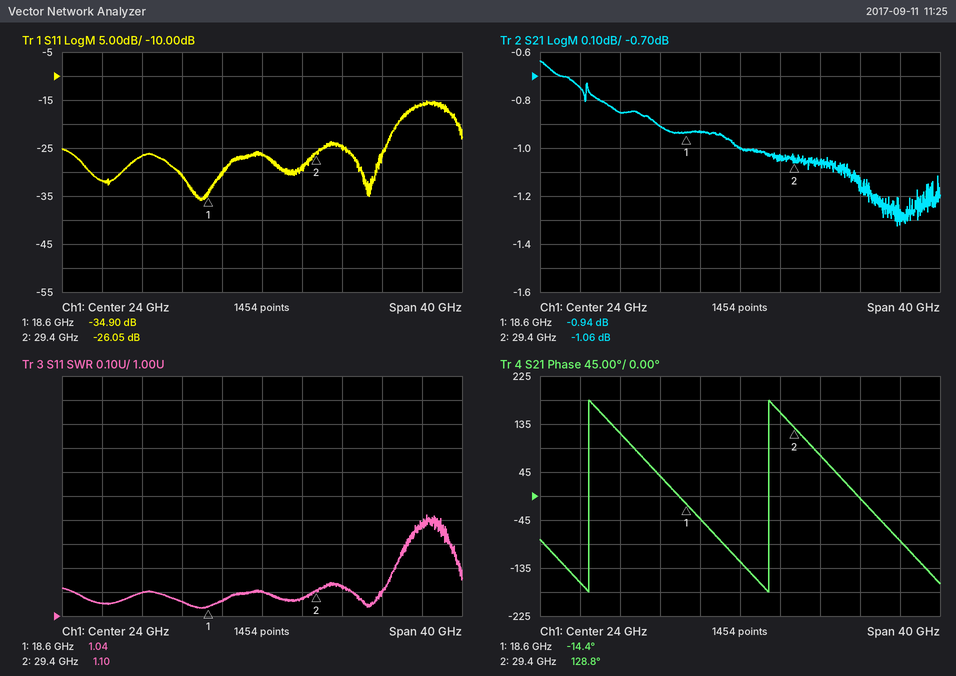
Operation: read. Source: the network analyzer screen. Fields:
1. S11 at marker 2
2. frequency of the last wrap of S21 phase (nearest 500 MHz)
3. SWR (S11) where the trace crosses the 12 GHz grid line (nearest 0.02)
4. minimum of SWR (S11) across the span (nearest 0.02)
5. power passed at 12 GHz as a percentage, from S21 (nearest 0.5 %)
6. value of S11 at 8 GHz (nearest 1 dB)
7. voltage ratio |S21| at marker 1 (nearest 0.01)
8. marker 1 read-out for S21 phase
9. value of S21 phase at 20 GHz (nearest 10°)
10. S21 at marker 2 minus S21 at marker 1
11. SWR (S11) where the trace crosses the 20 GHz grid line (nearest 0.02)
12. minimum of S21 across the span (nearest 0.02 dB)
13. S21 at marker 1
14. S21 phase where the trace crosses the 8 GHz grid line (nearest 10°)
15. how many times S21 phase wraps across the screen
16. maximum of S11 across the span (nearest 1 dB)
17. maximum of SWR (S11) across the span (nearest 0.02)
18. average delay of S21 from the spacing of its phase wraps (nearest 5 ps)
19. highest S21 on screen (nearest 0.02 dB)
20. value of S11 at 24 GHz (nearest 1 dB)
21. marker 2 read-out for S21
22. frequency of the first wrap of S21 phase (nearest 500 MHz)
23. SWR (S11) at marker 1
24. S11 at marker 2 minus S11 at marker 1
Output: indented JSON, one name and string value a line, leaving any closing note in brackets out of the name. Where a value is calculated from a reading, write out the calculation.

{
  "S11 at marker 2": "-26.05 dB",
  "frequency of the last wrap of S21 phase": "27.0 GHz",
  "SWR (S11) where the trace crosses the 12 GHz grid line": "1.10",
  "minimum of SWR (S11) across the span": "1.04",
  "power passed at 12 GHz as a percentage, from S21": "10^(-0.86/10) ≈ 82.0 %",
  "value of S11 at 8 GHz": "-32 dB",
  "voltage ratio |S21| at marker 1": "10^(-0.94/20) ≈ 0.90",
  "marker 1 read-out for S21 phase": "-14.4°",
  "value of S21 phase at 20 GHz": "-40°",
  "S21 at marker 2 minus S21 at marker 1": "-1.06 − (-0.94) = -0.12 dB",
  "SWR (S11) where the trace crosses the 20 GHz grid line": "1.06",
  "minimum of S21 across the span": "-1.32 dB",
  "S21 at marker 1": "-0.94 dB",
  "S21 phase where the trace crosses the 8 GHz grid line": "-160°",
  "how many times S21 phase wraps across the screen": "2",
  "maximum of S11 across the span": "-15 dB",
  "maximum of SWR (S11) across the span": "1.42",
  "average delay of S21 from the spacing of its phase wraps": "1 cycle / (27.0 GHz − 9.0 GHz) ≈ 55.6 ps, so 55 ps to the nearest 5 ps",
  "highest S21 on screen": "-0.64 dB",
  "value of S11 at 24 GHz": "-26 dB",
  "marker 2 read-out for S21": "-1.06 dB",
  "frequency of the first wrap of S21 phase": "9.0 GHz",
  "SWR (S11) at marker 1": "1.04",
  "S11 at marker 2 minus S11 at marker 1": "-26.05 − (-34.9) = 8.85 dB"
}
